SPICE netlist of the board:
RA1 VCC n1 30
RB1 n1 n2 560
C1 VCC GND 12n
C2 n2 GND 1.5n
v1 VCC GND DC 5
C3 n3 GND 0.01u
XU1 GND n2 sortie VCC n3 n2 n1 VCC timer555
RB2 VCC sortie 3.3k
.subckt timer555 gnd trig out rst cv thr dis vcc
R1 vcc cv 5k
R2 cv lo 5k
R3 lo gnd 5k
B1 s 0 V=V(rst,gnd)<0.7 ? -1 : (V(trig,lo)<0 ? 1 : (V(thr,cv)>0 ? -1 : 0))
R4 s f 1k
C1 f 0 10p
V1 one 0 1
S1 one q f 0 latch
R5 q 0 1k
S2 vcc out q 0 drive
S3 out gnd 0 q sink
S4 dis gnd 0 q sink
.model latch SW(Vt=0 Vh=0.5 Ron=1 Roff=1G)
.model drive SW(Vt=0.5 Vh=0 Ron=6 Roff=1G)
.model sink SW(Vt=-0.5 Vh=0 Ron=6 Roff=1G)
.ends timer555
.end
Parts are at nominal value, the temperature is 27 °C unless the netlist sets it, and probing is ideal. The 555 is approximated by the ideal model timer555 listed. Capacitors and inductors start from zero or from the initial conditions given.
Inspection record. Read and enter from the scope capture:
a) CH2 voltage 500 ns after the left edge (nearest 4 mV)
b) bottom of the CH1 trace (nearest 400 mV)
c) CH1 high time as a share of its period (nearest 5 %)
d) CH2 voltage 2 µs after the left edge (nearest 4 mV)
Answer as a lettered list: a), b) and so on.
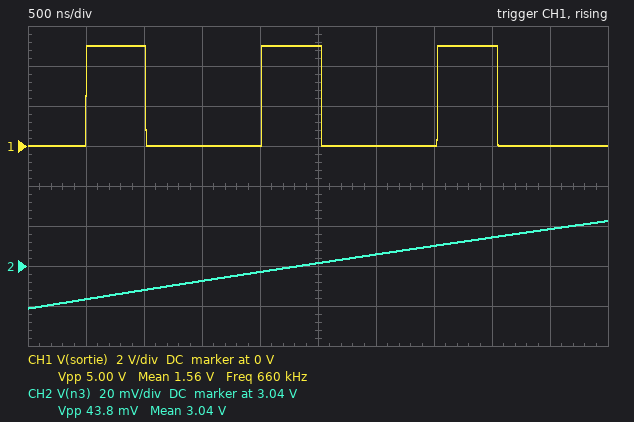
a) 3.024 V
b) 0 V
c) 35 %
d) 3.036 V
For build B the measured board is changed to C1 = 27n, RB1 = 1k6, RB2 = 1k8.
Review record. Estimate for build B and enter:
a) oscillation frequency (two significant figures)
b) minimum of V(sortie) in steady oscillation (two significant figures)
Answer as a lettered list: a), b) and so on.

a) 240 kHz
b) 17 mV
